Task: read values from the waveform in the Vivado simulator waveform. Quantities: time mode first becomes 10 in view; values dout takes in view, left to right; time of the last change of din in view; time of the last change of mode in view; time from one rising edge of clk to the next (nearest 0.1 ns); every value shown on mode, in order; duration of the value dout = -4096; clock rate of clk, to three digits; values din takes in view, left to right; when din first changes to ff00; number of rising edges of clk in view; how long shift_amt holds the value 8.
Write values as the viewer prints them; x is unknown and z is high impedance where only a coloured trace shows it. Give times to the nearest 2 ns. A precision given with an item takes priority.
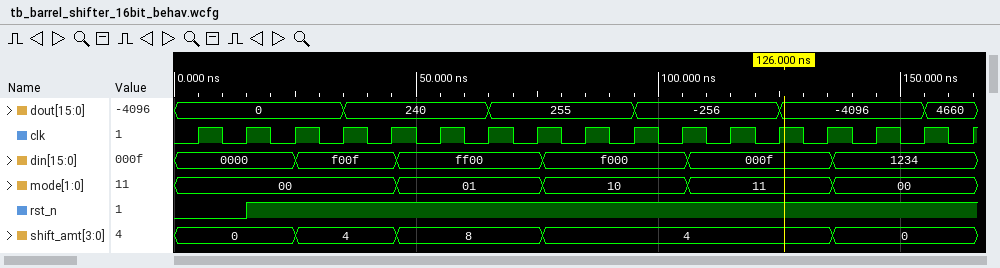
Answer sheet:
76 ns
0, 240, 255, -256, -4096, 4660
136 ns
136 ns
10 ns
00, 01, 10, 11, 00
30 ns
100 MHz
0000, f00f, ff00, f000, 000f, 1234
46 ns
17
30 ns
